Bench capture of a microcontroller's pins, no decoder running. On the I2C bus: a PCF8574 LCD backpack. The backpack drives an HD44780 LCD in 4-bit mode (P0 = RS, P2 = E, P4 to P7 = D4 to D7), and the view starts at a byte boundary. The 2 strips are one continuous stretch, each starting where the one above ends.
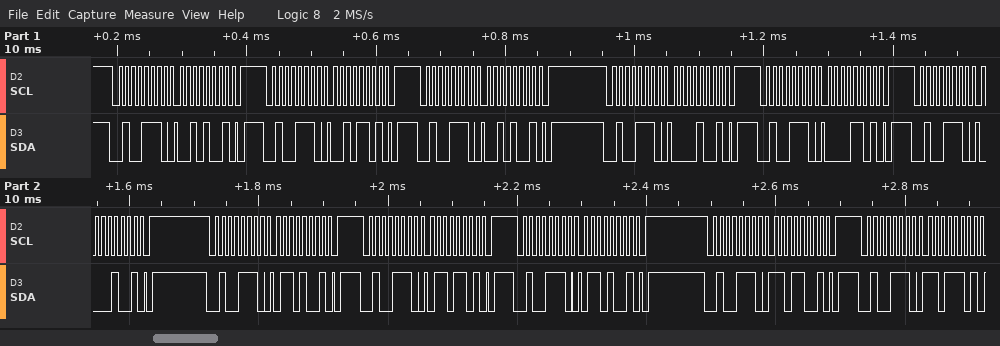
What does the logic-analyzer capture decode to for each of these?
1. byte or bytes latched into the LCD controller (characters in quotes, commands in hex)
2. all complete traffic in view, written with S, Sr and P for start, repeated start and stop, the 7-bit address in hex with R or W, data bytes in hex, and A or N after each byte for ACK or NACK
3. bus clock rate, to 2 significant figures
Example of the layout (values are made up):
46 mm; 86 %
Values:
' '; S 27W A 29 A P S 27W A 2D A P S 27W A 29 A P S 27W A 09 A P S 27W A 0D A P S 27W A 09 A P S 27W A 69 A P S 27W A 6D A P S 27W A 69 A P S 27W A D9 A P S 27W A DD A; 100 kHz
